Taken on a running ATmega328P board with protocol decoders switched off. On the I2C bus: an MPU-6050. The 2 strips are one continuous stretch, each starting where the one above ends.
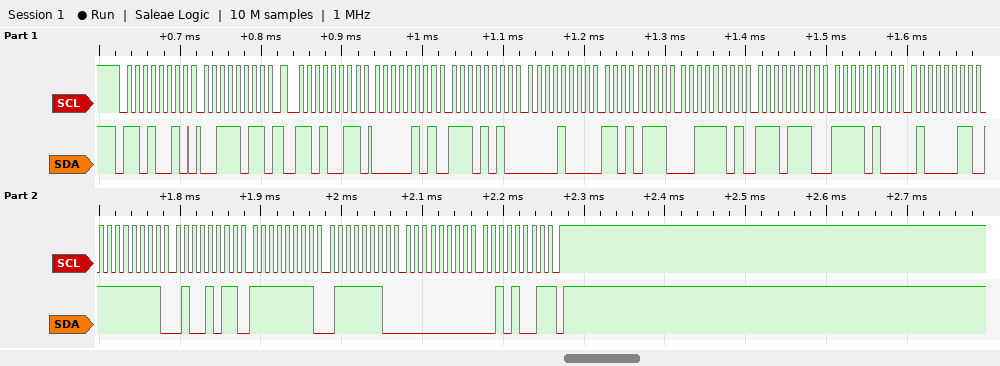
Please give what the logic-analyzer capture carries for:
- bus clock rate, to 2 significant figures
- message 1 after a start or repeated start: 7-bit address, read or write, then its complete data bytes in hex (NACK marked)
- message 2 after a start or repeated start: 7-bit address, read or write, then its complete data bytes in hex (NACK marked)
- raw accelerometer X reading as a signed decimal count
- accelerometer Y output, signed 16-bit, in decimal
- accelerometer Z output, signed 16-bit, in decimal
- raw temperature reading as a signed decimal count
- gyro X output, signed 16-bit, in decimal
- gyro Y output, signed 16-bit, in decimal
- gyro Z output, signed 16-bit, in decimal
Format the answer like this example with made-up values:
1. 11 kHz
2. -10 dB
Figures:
1. 100 kHz
2. 0x69 write: 3B
3. 0x69 read: 05 EA 08 D7 3D EE F4 43 FF 4B FF 7E 00 29 NACK
4. 1514
5. 2263
6. 15854
7. -3005
8. -181
9. -130
10. 41
